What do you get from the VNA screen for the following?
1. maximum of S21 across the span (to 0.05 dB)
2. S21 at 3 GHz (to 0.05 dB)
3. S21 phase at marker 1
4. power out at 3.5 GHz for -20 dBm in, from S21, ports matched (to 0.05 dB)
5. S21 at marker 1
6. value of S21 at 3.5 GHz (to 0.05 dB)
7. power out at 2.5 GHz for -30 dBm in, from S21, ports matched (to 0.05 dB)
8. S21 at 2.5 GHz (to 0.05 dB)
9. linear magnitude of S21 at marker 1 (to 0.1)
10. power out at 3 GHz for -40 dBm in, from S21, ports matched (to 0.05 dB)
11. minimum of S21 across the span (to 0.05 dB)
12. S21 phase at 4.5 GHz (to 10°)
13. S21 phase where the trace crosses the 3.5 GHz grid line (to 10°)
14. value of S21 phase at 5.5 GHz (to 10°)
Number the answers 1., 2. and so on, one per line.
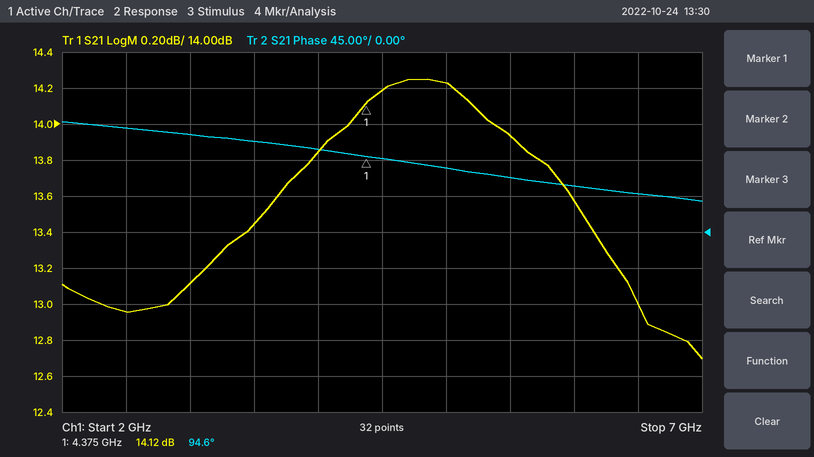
1. 14.25 dB
2. 13.10 dB
3. 94.6°
4. -6.55 dBm
5. 14.12 dB
6. 13.45 dB
7. -17.05 dBm
8. 12.95 dB
9. 5.1
10. -26.90 dBm
11. 12.70 dB
12. 90°
13. 110°
14. 70°
